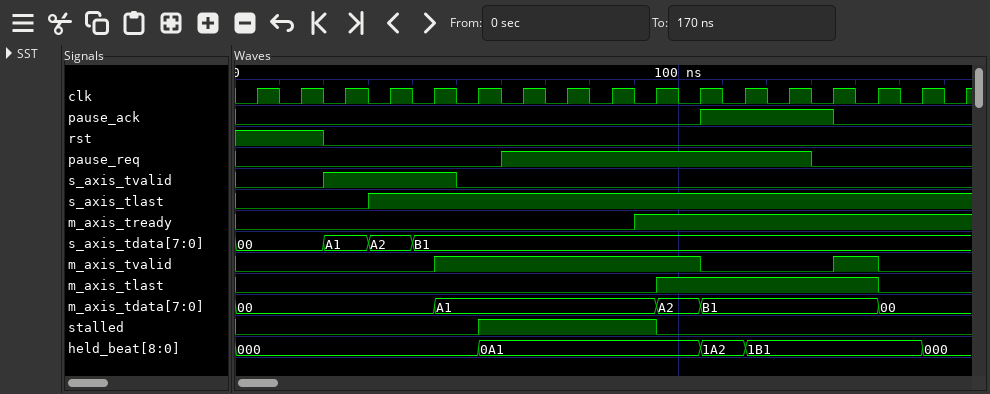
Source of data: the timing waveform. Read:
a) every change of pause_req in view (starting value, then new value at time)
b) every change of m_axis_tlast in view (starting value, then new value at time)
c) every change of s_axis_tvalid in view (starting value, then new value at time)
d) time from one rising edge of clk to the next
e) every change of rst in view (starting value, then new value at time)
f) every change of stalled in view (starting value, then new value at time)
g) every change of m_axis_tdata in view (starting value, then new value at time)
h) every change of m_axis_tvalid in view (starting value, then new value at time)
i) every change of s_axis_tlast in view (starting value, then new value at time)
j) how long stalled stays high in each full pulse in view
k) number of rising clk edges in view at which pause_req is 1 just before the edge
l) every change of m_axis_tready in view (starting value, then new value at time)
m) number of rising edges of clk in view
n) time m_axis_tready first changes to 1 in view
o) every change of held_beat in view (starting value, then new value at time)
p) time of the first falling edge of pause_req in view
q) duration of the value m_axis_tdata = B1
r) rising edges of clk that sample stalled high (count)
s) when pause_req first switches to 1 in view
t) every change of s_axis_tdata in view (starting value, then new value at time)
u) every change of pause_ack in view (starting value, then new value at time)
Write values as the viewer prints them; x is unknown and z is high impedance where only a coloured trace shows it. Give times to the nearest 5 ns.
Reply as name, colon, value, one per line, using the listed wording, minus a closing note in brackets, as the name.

every change of pause_req in view: 0, 1 at 60 ns, 0 at 130 ns
every change of m_axis_tlast in view: 0, 1 at 95 ns, 0 at 145 ns
every change of s_axis_tvalid in view: 0, 1 at 20 ns, 0 at 50 ns
time from one rising edge of clk to the next: 10 ns
every change of rst in view: 1, 0 at 20 ns
every change of stalled in view: 0, 1 at 55 ns, 0 at 95 ns
every change of m_axis_tdata in view: 00, A1 at 45 ns, A2 at 95 ns, B1 at 105 ns, 00 at 145 ns
every change of m_axis_tvalid in view: 0, 1 at 45 ns, 0 at 105 ns, 1 at 135 ns, 0 at 145 ns
every change of s_axis_tlast in view: 0, 1 at 30 ns
how long stalled stays high in each full pulse in view: 40 ns
number of rising clk edges in view at which pause_req is 1 just before the edge: 7
every change of m_axis_tready in view: 0, 1 at 90 ns
number of rising edges of clk in view: 17
time m_axis_tready first changes to 1 in view: 90 ns
every change of held_beat in view: 000, 0A1 at 55 ns, 1A2 at 105 ns, 1B1 at 115 ns, 000 at 155 ns
time of the first falling edge of pause_req in view: 130 ns
duration of the value m_axis_tdata = B1: 40 ns
rising edges of clk that sample stalled high: 4
when pause_req first switches to 1 in view: 60 ns
every change of s_axis_tdata in view: 00, A1 at 20 ns, A2 at 30 ns, B1 at 40 ns
every change of pause_ack in view: 0, 1 at 105 ns, 0 at 135 ns
